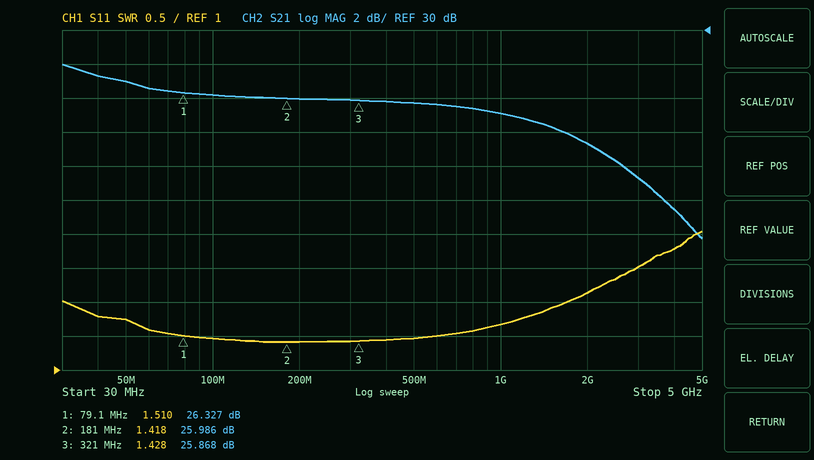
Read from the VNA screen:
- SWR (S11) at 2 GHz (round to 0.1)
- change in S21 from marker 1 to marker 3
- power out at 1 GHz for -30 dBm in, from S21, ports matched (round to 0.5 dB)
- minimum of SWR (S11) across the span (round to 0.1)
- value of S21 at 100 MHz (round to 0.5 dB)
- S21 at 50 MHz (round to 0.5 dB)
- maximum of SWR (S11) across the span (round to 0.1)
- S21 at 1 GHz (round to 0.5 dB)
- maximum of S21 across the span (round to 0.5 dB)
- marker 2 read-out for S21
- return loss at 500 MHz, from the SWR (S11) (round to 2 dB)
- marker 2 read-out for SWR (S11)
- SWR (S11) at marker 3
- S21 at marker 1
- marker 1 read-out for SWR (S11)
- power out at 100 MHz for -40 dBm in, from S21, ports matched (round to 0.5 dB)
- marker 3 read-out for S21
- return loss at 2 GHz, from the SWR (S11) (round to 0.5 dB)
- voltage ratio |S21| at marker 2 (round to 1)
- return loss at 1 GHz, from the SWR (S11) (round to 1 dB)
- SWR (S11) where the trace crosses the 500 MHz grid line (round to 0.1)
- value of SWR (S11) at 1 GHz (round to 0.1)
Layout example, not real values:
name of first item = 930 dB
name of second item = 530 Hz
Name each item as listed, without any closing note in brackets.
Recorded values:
SWR (S11) at 2 GHz = 2.1
change in S21 from marker 1 to marker 3 = -0.459 dB
power out at 1 GHz for -30 dBm in, from S21, ports matched = -5.0 dBm
minimum of SWR (S11) across the span = 1.4
value of S21 at 100 MHz = 26.0 dB
S21 at 50 MHz = 27.0 dB
maximum of SWR (S11) across the span = 3.0
S21 at 1 GHz = 25.0 dB
maximum of S21 across the span = 28.0 dB
marker 2 read-out for S21 = 25.986 dB
return loss at 500 MHz, from the SWR (S11) = 14 dB
marker 2 read-out for SWR = 1.418
SWR (S11) at marker 3 = 1.428
S21 at marker 1 = 26.327 dB
marker 1 read-out for SWR = 1.510
power out at 100 MHz for -40 dBm in, from S21, ports matched = -14.0 dBm
marker 3 read-out for S21 = 25.868 dB
return loss at 2 GHz, from the SWR (S11) = 9.0 dB
voltage ratio |S21| at marker 2 = 20
return loss at 1 GHz, from the SWR (S11) = 12 dB
SWR (S11) where the trace crosses the 500 MHz grid line = 1.5
value of SWR (S11) at 1 GHz = 1.7
